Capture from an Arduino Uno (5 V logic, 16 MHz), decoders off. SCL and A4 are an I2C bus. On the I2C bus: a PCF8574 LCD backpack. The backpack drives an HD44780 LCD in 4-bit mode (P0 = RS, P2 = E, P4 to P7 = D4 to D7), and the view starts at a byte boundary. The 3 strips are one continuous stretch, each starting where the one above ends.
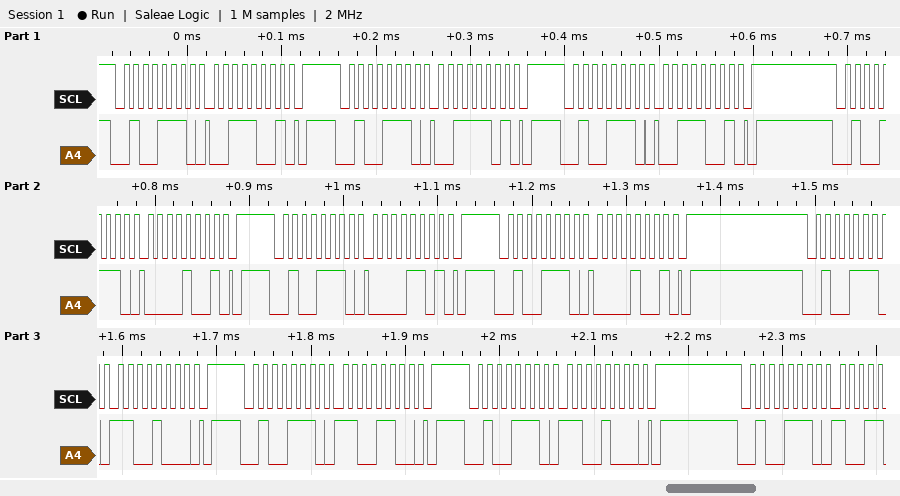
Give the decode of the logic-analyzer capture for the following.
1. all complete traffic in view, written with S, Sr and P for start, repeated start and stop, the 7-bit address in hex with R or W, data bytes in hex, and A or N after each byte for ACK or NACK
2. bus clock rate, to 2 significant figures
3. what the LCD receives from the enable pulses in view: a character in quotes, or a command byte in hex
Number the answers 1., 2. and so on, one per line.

1. S 27W A 39 A P S 27W A 3D A P S 27W A 39 A P S 27W A 09 A P S 27W A 0D A P S 27W A 09 A P S 27W A C8 A P S 27W A CC A P S 27W A C8 A P S 27W A
2. 100 kHz
3. '0'
